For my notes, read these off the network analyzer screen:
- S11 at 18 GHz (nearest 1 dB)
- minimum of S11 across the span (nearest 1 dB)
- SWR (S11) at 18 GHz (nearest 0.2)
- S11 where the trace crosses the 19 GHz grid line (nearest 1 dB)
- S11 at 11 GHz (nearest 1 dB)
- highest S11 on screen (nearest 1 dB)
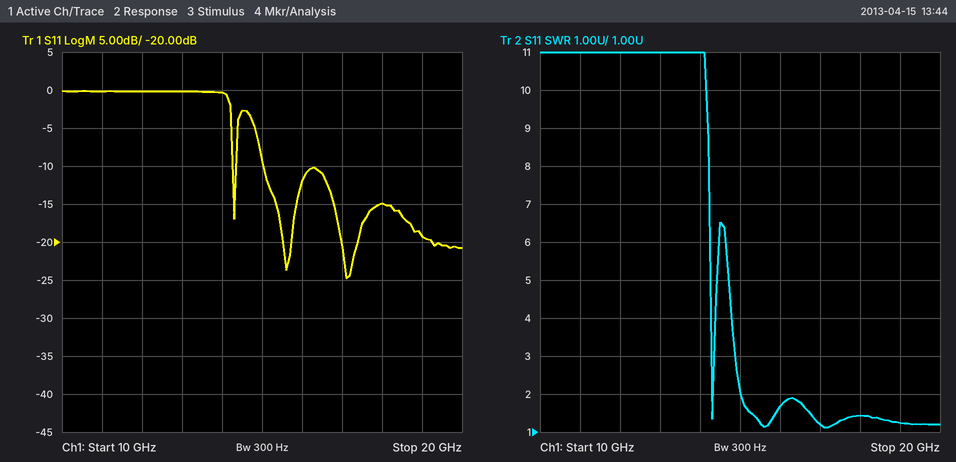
-15 dB
-25 dB
1.4
-19 dB
0 dB
0 dB
